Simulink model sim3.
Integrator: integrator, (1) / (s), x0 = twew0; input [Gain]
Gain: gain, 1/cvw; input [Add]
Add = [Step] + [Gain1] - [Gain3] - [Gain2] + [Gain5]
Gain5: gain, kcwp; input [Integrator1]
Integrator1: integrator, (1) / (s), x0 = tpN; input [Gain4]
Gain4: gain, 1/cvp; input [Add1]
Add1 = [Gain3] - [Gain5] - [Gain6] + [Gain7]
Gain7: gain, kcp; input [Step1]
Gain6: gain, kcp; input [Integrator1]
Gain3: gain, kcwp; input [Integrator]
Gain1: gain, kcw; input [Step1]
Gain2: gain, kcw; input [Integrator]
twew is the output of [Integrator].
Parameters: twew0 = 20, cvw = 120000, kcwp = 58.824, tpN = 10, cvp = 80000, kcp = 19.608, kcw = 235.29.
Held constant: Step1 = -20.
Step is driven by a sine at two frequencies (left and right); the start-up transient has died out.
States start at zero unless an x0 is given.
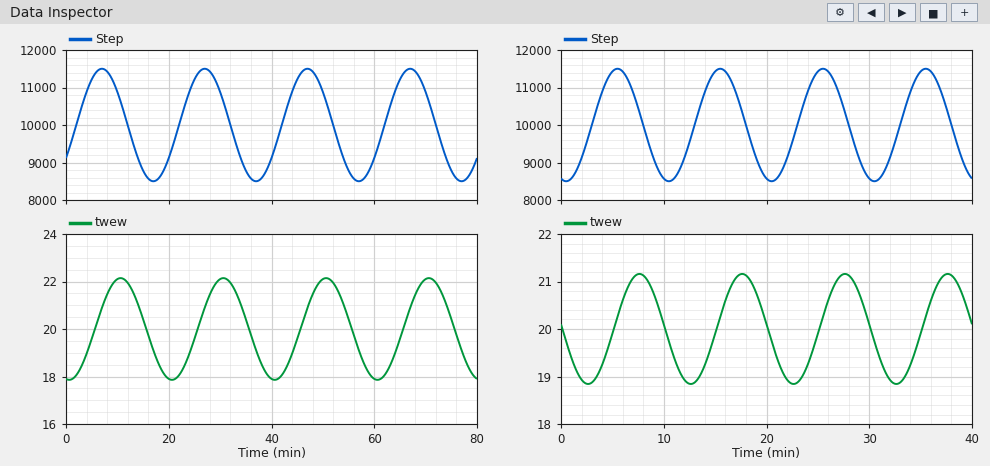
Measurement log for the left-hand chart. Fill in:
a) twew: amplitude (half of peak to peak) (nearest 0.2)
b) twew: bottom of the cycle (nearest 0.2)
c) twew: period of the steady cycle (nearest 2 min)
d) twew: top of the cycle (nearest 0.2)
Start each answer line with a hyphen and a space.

- 2.2
- 17.8
- 20 min
- 22.2
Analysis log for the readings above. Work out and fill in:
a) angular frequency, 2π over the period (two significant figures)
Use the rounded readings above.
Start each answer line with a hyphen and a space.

- 0.31 rad/min
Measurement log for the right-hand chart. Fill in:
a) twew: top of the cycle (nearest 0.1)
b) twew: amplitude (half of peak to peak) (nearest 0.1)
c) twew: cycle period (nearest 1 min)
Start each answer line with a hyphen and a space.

- 21.2
- 1.2
- 10 min
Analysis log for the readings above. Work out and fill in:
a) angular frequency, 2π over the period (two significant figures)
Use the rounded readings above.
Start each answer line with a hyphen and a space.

- 0.63 rad/min
